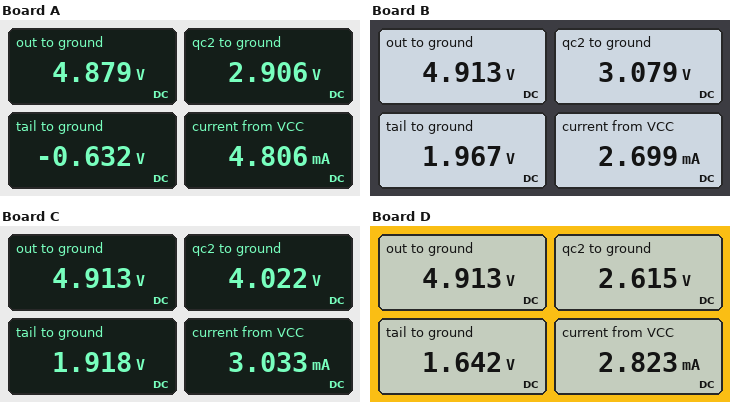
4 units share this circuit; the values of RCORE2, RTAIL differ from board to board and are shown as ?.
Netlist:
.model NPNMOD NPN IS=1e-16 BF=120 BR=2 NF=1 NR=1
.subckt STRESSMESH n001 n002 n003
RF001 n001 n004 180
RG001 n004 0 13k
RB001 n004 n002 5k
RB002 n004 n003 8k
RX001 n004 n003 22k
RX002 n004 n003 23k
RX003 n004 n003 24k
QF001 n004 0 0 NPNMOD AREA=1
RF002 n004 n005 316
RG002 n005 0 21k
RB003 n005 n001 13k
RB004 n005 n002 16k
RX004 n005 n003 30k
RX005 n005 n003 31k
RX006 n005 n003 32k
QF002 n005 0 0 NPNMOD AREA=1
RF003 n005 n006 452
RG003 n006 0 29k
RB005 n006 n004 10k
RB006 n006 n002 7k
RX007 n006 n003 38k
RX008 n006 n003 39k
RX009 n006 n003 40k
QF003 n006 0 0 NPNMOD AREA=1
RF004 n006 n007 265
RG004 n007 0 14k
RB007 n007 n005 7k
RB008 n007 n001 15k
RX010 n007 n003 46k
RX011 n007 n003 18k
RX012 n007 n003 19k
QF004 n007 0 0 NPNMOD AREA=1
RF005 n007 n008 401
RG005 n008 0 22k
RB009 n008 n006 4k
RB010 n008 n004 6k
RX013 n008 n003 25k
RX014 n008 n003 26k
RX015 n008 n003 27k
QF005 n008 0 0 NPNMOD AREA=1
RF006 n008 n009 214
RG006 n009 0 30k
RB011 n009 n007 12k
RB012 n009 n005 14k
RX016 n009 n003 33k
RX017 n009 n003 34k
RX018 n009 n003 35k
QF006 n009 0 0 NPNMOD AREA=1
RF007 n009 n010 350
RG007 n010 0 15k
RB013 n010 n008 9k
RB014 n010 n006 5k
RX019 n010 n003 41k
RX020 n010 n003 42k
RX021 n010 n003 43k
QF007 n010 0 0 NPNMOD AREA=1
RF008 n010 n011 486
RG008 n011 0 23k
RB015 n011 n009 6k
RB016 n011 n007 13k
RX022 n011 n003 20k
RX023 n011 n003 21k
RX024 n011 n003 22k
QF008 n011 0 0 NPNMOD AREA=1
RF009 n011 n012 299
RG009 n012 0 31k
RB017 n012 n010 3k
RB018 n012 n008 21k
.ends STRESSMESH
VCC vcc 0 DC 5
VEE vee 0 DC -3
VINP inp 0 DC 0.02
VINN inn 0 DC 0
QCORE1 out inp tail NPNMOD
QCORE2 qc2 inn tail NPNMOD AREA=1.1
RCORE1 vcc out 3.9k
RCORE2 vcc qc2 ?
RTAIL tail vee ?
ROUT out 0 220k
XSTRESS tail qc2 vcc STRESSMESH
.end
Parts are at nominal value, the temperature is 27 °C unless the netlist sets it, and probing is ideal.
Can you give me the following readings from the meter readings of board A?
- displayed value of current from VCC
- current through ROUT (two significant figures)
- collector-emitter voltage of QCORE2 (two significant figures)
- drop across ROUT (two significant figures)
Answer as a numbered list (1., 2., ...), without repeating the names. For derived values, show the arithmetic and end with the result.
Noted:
1. 4.806 mA
2. (4.879 V) / 220 kΩ = 22 µA
3. 2.906 V - (-632 mV) = 3.5 V
4. 4.879 V = 4.9 V
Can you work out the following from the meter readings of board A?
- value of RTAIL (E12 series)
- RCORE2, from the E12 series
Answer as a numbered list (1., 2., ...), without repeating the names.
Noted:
1. 560 Ω
2. 2.2 kΩ
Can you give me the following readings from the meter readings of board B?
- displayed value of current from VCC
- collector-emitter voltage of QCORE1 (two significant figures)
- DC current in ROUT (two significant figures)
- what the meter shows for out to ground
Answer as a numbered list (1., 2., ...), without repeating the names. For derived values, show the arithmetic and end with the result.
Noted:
1. 2.699 mA
2. 4.913 V - 1.967 V = 2.9 V
3. (4.913 V) / 220 kΩ = 22 µA
4. 4.913 V
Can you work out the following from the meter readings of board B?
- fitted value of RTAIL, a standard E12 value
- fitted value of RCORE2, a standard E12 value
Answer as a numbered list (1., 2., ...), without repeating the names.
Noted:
1. 3.3 kΩ
2. 6.8 kΩ
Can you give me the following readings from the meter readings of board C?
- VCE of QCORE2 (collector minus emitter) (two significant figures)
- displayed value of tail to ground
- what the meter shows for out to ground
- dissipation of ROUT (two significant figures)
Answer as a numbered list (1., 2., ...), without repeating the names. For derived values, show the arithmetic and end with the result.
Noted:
1. 4.022 V - 1.918 V = 2.1 V
2. 1.918 V
3. 4.913 V
4. (4.913 V)^2 / 220 kΩ = 110 µW
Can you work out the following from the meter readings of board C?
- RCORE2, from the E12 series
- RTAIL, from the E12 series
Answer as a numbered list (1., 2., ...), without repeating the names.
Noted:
1. 1.5 kΩ
2. 2.7 kΩ
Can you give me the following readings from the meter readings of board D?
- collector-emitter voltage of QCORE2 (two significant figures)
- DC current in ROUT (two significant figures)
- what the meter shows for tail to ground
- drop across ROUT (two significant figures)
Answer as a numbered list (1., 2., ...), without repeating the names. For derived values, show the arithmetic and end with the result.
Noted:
1. 2.615 V - 1.642 V = 970 mV
2. (4.913 V) / 220 kΩ = 22 µA
3. 1.642 V
4. 4.913 V = 4.9 V
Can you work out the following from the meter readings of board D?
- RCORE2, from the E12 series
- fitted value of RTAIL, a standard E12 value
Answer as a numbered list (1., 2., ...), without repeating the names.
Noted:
1. 12 kΩ
2. 2.7 kΩ
